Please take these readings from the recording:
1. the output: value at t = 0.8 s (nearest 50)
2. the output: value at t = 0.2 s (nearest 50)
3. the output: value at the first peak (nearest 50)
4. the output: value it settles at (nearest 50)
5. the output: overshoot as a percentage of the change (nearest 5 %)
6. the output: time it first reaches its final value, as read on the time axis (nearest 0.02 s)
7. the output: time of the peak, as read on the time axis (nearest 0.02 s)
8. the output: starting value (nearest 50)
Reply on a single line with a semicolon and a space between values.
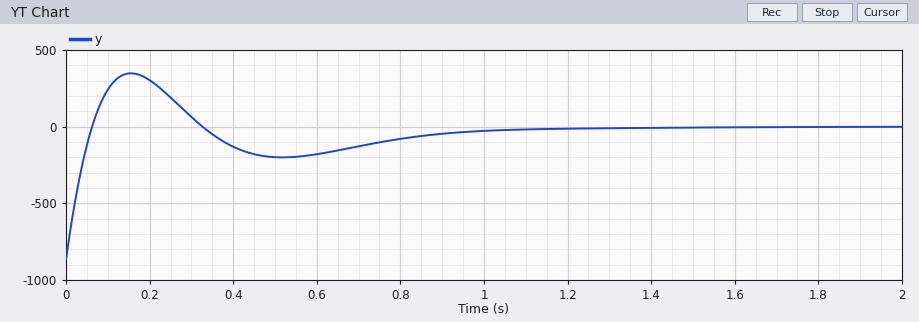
-100; 300; 350; 0; 40 %; 0.06 s; 0.16 s; -850
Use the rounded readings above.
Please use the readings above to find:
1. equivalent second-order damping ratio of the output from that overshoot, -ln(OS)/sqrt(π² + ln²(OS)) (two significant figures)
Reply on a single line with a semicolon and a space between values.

0.28
